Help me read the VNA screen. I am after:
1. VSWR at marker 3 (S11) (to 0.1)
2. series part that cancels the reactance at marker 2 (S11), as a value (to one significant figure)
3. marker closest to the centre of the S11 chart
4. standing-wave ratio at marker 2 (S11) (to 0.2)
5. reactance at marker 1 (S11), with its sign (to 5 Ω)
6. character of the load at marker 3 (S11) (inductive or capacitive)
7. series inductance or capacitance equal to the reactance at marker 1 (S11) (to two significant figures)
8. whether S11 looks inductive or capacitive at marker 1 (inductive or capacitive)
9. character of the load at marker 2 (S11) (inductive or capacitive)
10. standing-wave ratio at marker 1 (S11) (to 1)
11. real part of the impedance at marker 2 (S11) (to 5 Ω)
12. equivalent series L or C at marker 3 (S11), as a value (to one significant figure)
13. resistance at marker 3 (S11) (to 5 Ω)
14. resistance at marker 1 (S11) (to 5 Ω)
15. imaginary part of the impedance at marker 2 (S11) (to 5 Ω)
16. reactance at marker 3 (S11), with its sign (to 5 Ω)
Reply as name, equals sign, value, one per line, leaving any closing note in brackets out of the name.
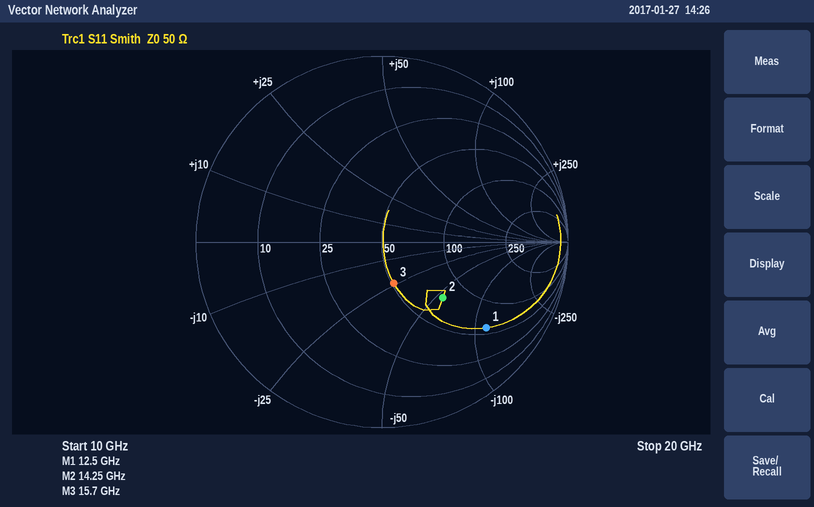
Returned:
VSWR at marker 3 (S11) = 1.6
series part that cancels the reactance at marker 2 (S11), as a value = 600 pH
marker closest to the centre of the S11 chart = marker 3
standing-wave ratio at marker 2 (S11) = 2.6
reactance at marker 1 (S11), with its sign = -115 Ω
character of the load at marker 3 (S11) = capacitive
series inductance or capacitance equal to the reactance at marker 1 (S11) = 110 fF
whether S11 looks inductive or capacitive at marker 1 = capacitive
character of the load at marker 2 (S11) = capacitive
standing-wave ratio at marker 1 (S11) = 6
real part of the impedance at marker 2 (S11) = 75 Ω
equivalent series L or C at marker 3 (S11), as a value = 400 fF
resistance at marker 3 (S11) = 50 Ω
resistance at marker 1 (S11) = 60 Ω
imaginary part of the impedance at marker 2 (S11) = -55 Ω
reactance at marker 3 (S11), with its sign = -25 Ω
